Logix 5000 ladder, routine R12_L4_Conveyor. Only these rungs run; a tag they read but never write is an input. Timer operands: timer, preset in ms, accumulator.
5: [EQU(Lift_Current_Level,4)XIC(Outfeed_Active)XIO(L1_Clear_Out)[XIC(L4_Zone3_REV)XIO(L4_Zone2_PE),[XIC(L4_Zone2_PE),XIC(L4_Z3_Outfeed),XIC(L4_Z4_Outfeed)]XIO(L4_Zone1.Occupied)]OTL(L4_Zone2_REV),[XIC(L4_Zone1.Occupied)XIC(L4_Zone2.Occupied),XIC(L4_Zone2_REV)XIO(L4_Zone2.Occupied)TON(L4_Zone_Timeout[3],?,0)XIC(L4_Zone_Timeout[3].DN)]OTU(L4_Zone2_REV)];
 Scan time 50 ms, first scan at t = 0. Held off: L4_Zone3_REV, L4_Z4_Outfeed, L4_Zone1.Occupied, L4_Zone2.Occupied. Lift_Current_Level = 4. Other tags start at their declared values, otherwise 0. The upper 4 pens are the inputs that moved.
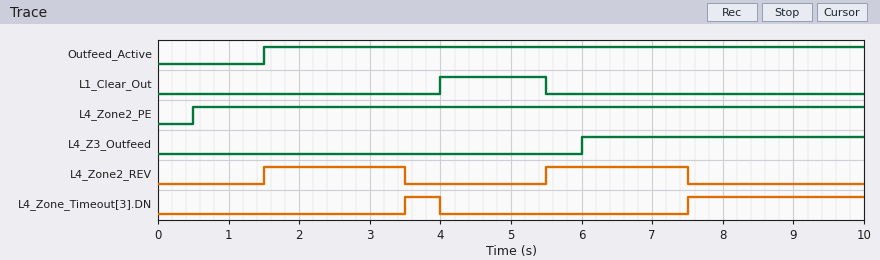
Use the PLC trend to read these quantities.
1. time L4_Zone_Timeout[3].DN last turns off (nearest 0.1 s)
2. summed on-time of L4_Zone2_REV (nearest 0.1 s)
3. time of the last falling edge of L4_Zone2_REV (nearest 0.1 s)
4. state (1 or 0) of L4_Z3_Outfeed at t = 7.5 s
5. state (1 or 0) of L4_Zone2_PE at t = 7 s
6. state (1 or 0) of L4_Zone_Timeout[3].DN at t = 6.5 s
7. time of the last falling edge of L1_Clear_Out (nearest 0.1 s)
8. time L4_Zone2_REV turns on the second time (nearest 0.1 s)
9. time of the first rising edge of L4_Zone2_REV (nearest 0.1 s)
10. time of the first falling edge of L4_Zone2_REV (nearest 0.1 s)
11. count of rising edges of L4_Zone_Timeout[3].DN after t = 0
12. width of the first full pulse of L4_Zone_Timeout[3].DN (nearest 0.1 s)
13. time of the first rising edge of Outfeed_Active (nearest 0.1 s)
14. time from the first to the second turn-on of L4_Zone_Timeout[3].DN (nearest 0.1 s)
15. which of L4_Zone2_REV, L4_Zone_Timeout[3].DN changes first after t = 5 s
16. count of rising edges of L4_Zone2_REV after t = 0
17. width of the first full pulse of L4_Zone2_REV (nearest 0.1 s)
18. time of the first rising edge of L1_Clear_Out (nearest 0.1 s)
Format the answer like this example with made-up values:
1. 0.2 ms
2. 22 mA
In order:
1. 4.0 s
2. 4.0 s
3. 7.5 s
4. 1
5. 1
6. 0
7. 5.5 s
8. 5.5 s
9. 1.5 s
10. 3.5 s
11. 2
12. 0.5 s
13. 1.5 s
14. 4.0 s
15. L4_Zone2_REV
16. 2
17. 2.0 s
18. 4.0 s
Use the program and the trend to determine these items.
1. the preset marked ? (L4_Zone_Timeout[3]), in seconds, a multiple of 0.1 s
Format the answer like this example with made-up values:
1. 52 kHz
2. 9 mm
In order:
1. 2.0 s
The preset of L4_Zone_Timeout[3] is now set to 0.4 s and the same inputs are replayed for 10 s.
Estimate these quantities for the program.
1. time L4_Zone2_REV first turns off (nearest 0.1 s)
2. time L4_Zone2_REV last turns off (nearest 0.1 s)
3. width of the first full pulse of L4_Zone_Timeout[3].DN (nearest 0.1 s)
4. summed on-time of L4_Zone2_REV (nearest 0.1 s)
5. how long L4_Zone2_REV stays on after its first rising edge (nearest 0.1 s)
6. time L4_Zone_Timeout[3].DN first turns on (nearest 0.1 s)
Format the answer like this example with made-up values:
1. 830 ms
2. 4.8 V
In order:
1. 1.9 s
2. 5.9 s
3. 2.1 s
4. 0.8 s
5. 0.4 s
6. 1.9 s
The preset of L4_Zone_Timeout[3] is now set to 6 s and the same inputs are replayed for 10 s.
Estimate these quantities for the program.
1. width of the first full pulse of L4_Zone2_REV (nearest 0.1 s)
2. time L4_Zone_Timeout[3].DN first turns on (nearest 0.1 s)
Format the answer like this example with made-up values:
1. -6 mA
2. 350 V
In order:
1. 6.0 s
2. 7.5 s
